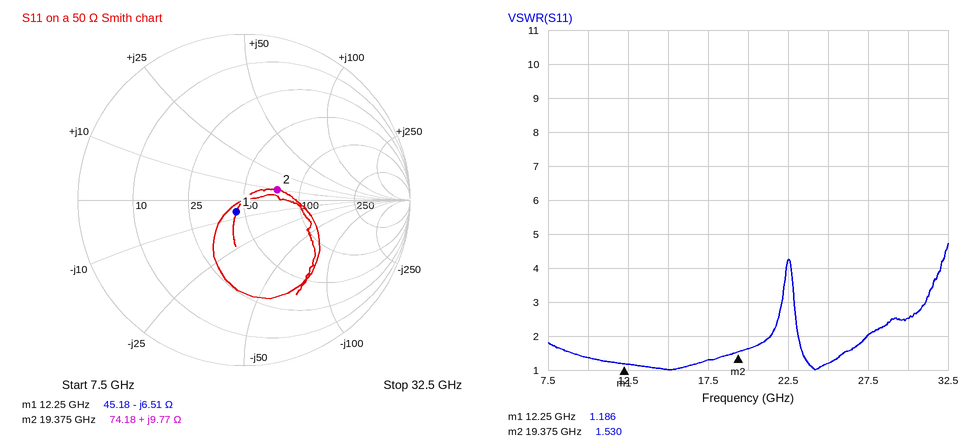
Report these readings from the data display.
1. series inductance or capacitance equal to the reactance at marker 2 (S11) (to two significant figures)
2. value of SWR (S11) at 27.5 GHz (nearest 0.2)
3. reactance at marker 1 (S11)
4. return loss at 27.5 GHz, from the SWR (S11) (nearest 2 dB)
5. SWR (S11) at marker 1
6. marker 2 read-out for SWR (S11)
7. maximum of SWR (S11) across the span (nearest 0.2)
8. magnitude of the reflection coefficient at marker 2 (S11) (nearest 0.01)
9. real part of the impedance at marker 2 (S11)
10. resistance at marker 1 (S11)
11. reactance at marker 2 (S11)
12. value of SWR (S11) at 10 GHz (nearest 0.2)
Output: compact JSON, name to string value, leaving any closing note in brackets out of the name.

{"series inductance or capacitance equal to the reactance at marker 2 (S11)": "80 pH", "value of SWR (S11) at 27.5 GHz": "2.0", "reactance at marker 1": "-6.51 Ω", "return loss at 27.5 GHz, from the SWR (S11)": "10 dB", "SWR (S11) at marker 1": "1.186", "marker 2 read-out for SWR": "1.530", "maximum of SWR (S11) across the span": "4.8", "magnitude of the reflection coefficient at marker 2 (S11)": "0.21", "real part of the impedance at marker 2": "74.18 Ω", "resistance at marker 1": "45.18 Ω", "reactance at marker 2": "+9.77 Ω", "value of SWR (S11) at 10 GHz": "1.4"}
